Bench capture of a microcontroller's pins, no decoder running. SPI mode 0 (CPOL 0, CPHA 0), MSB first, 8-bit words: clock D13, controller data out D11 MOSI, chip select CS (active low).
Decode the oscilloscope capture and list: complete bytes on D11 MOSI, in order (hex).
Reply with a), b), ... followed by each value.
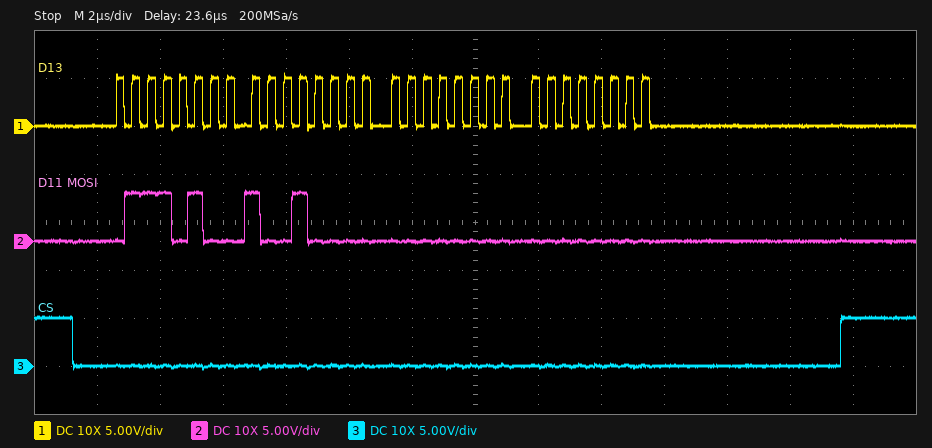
a) 74 90 00 00
